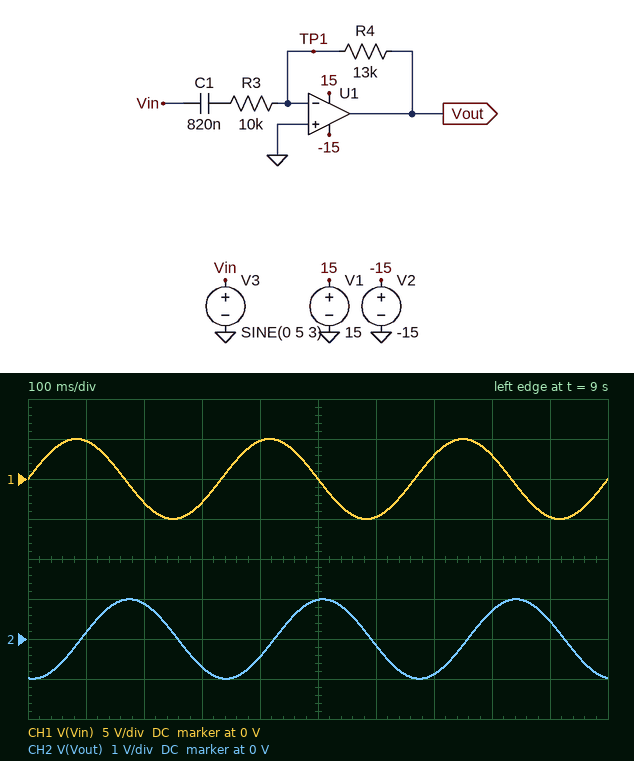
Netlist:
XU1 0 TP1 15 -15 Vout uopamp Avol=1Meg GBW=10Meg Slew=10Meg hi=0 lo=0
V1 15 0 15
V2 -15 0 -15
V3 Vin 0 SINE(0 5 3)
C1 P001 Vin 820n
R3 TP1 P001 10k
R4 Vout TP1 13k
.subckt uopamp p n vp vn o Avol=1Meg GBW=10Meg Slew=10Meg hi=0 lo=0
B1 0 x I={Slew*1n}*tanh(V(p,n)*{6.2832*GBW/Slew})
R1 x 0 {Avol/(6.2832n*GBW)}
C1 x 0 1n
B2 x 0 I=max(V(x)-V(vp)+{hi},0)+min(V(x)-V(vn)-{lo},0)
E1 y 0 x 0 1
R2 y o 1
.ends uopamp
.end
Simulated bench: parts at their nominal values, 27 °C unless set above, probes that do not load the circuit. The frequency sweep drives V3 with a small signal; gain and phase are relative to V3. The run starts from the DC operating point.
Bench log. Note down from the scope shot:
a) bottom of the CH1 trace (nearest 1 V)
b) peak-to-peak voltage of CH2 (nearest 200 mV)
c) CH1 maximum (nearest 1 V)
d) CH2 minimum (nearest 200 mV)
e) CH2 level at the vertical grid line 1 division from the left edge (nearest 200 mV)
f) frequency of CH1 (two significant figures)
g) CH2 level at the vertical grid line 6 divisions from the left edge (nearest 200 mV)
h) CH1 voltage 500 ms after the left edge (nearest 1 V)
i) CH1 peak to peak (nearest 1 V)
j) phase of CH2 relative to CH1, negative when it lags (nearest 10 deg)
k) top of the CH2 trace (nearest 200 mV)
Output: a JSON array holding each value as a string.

["-5 V", "2.0 V", "5 V", "-1.0 V", "200 mV", "3.0 Hz", "-200 mV", "0 V", "10 V", "-100 deg", "1.0 V"]
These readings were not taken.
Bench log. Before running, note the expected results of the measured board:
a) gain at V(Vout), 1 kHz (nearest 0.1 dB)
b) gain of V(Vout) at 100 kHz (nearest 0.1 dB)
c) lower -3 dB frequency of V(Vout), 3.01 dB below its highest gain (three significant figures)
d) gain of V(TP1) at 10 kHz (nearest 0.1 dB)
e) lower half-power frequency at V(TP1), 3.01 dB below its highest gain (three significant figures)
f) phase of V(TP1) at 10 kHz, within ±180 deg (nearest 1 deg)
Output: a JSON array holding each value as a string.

["2.3 dB", "2.3 dB", "19.4 Hz", "-57.7 dB", "4.35 MHz", "90 deg"]
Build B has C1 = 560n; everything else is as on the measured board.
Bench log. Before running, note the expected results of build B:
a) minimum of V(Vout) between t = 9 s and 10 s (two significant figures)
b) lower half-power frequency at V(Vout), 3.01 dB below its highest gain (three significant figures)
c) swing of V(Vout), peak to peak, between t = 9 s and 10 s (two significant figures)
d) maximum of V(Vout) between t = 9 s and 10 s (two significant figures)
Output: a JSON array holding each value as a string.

["-680 mV", "28.4 Hz", "1.4 V", "680 mV"]
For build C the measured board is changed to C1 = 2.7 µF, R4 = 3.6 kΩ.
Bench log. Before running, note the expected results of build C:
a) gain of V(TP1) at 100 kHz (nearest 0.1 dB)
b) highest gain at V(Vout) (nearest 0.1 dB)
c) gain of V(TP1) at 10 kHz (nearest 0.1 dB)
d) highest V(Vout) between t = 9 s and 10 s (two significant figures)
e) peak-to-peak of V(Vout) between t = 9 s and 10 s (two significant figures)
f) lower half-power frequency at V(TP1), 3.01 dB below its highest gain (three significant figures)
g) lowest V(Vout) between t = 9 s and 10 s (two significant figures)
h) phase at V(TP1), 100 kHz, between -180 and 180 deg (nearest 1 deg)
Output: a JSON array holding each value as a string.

["-48.9 dB", "-8.9 dB", "-68.9 dB", "820 mV", "1.6 V", "7.35 MHz", "-820 mV", "89 deg"]
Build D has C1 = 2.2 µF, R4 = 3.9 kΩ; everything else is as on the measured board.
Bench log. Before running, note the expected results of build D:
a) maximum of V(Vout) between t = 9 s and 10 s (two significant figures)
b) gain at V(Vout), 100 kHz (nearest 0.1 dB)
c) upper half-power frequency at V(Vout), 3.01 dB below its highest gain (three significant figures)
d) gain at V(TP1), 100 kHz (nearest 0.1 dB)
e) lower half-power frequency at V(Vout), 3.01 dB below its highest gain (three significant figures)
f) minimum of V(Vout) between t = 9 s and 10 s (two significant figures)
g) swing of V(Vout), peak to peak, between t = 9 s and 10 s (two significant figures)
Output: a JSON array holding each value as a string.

["750 mV", "-8.2 dB", "7.19 MHz", "-48.2 dB", "7.23 Hz", "-750 mV", "1.5 V"]
